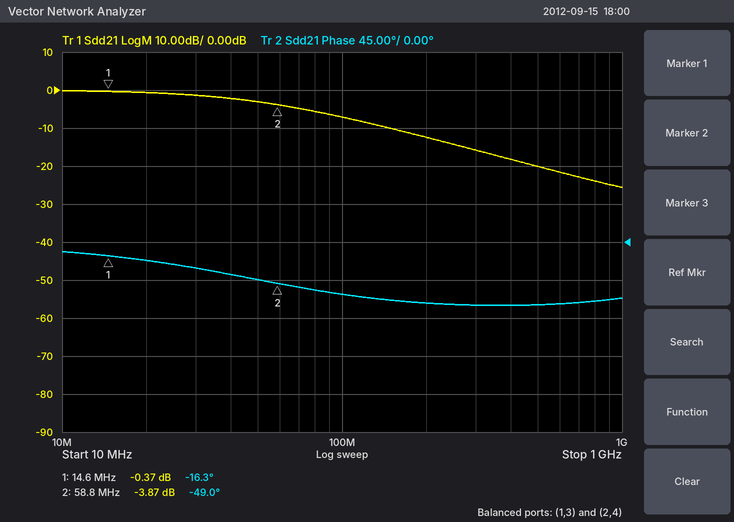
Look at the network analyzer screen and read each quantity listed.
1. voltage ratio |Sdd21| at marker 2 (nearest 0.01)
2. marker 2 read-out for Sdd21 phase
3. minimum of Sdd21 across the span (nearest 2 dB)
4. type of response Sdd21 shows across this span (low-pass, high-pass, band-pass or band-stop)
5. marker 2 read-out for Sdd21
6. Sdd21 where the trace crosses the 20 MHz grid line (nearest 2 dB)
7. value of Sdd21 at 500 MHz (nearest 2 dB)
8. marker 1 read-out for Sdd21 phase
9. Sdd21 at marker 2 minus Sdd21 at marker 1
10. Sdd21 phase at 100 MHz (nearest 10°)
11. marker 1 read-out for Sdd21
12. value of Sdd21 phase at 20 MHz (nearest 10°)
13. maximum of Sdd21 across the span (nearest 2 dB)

0.64
-49.0°
-26 dB
low-pass
-3.87 dB
0 dB
-20 dB
-16.3°
-3.50 dB
-60°
-0.37 dB
-20°
0 dB
